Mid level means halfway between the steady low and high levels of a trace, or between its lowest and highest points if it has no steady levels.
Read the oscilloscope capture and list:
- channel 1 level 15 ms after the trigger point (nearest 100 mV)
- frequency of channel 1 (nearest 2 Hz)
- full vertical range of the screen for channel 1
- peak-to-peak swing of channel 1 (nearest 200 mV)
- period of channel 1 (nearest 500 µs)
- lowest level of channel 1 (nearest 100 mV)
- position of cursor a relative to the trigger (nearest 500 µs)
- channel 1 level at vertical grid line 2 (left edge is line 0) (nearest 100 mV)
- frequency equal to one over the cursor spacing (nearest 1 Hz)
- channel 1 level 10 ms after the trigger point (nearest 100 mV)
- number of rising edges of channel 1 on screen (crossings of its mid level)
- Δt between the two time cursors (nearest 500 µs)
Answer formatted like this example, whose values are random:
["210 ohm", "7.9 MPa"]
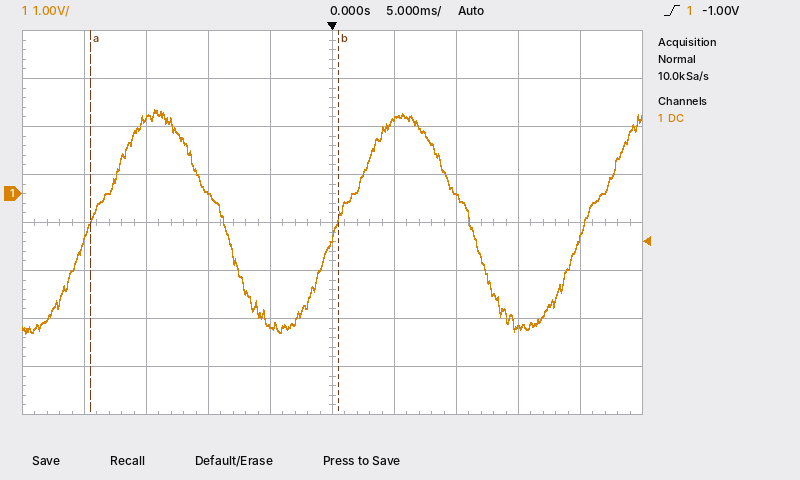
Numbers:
["-2.8 V", "50 Hz", "8 V", "4.6 V", "20.0 ms", "-2.9 V", "-19.5 ms", "1.6 V", "50 Hz", "0.0 V", "3", "20.0 ms"]
